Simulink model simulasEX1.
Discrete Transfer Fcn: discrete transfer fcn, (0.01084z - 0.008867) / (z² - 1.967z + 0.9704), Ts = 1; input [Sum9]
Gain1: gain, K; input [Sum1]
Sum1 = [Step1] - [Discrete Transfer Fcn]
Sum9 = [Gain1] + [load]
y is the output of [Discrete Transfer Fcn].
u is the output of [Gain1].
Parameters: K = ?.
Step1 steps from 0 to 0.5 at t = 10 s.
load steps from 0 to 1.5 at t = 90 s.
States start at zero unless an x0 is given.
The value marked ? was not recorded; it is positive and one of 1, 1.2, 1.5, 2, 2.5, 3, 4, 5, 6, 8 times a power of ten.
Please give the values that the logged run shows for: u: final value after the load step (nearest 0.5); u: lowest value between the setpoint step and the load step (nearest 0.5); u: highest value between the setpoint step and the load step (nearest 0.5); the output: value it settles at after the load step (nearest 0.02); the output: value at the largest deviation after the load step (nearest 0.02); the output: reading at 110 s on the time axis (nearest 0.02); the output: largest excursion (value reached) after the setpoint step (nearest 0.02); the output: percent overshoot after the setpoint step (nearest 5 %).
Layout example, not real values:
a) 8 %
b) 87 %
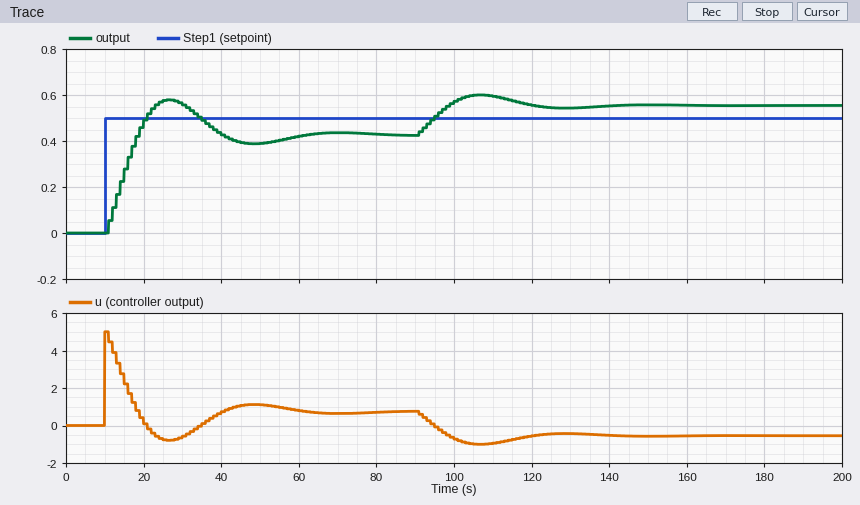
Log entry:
a) -0.5
b) -1.0
c) 5.0
d) 0.56
e) 0.60
f) 0.60
g) 0.58
h) 35 %
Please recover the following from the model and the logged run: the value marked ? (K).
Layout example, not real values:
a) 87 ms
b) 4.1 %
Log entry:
a) 10
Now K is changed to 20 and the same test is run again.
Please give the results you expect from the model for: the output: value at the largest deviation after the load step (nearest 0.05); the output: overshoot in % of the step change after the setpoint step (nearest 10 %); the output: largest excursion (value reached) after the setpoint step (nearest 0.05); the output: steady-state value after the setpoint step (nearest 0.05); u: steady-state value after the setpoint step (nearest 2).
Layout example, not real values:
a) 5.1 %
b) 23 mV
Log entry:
a) 0.55
b) 30 %
c) 0.60
d) 0.45
e) 0
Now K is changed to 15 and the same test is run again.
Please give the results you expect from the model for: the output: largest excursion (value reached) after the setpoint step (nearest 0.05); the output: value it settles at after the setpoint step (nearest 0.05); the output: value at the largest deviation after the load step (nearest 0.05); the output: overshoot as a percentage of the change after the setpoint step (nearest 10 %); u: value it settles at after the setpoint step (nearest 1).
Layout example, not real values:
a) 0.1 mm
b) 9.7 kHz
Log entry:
a) 0.60
b) 0.45
c) 0.55
d) 30 %
e) 1
